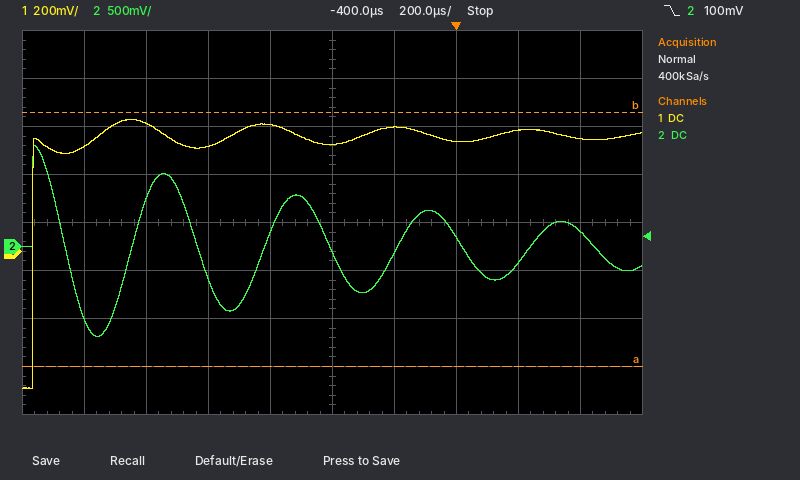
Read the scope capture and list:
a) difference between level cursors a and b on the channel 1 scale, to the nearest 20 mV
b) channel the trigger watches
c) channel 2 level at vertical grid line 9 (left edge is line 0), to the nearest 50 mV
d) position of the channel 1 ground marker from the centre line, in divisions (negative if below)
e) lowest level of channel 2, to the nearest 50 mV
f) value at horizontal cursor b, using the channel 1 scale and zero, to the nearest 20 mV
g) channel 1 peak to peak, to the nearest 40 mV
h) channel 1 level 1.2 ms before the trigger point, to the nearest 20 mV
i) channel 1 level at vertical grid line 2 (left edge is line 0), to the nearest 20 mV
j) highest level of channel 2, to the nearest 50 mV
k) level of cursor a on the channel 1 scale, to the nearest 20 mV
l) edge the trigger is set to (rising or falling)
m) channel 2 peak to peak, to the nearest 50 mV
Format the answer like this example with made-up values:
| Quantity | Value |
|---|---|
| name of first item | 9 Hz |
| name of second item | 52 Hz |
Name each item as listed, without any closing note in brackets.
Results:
| Quantity | Value |
|---|---|
| difference between level cursors a and b on the channel 1 scale, to the nearest 20 mV | 1.06 V |
| channel the trigger watches | channel 2 |
| channel 2 level at vertical grid line 9 (left edge is line 0), to the nearest 50 mV | 150 mV |
| position of the channel 1 ground marker from the centre line, in divisions | -0.6 div |
| lowest level of channel 2, to the nearest 50 mV | -950 mV |
| value at horizontal cursor b, using the channel 1 scale and zero, to the nearest 20 mV | 580 mV |
| channel 1 peak to peak, to the nearest 40 mV | 1.12 V |
| channel 1 level 1.2 ms before the trigger point, to the nearest 20 mV | 440 mV |
| channel 1 level at vertical grid line 2 (left edge is line 0), to the nearest 20 mV | 540 mV |
| highest level of channel 2, to the nearest 50 mV | 1.05 V |
| level of cursor a on the channel 1 scale, to the nearest 20 mV | -480 mV |
| edge the trigger is set to | falling |
| channel 2 peak to peak, to the nearest 50 mV | 2.00 V |
